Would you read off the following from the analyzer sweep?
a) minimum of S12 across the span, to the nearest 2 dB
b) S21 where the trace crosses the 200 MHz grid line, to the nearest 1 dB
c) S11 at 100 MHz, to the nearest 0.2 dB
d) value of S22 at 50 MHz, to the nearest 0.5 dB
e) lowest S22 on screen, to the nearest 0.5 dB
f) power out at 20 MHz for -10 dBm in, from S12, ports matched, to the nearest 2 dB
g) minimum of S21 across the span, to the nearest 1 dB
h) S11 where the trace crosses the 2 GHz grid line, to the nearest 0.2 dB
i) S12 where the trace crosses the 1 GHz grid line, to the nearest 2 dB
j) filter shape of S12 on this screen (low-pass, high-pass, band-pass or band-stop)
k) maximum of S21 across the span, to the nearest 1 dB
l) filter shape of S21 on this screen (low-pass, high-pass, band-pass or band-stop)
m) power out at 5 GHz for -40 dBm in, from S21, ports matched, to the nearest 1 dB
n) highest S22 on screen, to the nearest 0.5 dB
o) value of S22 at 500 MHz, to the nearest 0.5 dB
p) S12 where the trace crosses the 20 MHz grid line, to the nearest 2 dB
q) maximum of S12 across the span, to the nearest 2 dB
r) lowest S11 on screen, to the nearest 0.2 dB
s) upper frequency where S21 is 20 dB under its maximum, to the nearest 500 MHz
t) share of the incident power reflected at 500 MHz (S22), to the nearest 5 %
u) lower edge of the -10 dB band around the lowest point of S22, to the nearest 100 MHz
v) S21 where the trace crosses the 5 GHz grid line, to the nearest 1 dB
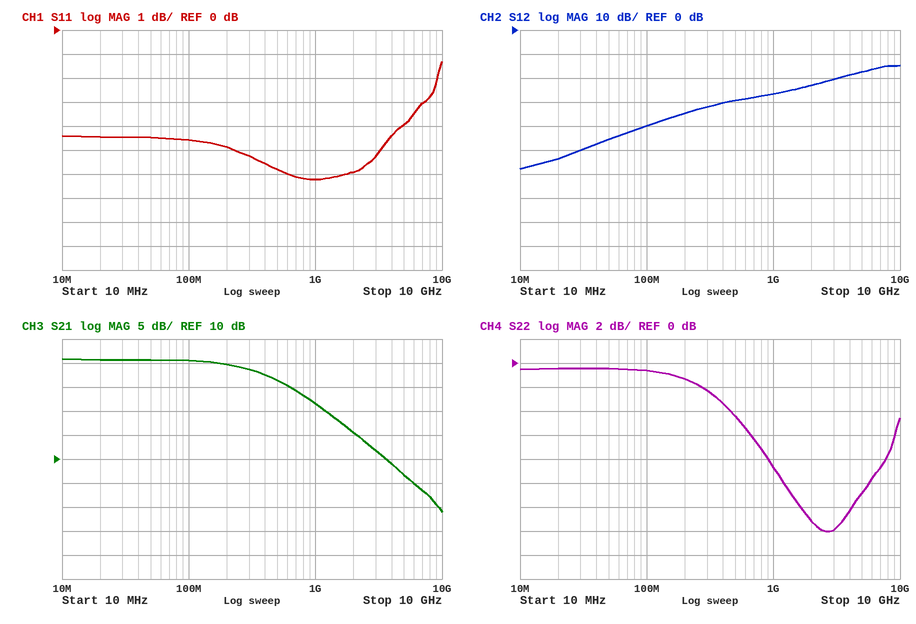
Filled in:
-58 dB
30 dB
-4.6 dB
-0.5 dB
-14.0 dB
-64 dBm
-1 dB
-6.0 dB
-26 dB
high-pass
31 dB
low-pass
-33 dBm
-0.5 dB
-4.5 dB
-54 dB
-14 dB
-6.2 dB
3.5 GHz
35 %
1.2 GHz
7 dB
